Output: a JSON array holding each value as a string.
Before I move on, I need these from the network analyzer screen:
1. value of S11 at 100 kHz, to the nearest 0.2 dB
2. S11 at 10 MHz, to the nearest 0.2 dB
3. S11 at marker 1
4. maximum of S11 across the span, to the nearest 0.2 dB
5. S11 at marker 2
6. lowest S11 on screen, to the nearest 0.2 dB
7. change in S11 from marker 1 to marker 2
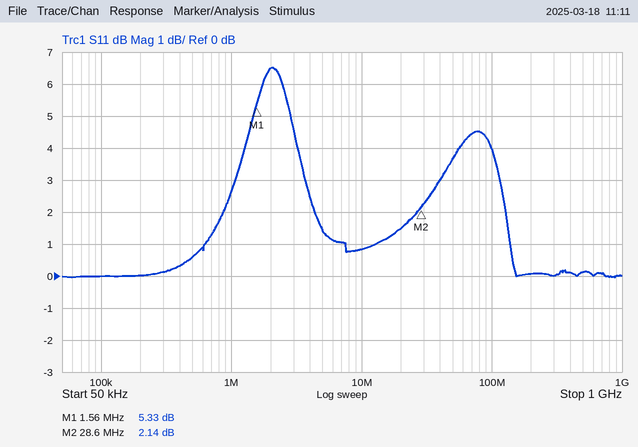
["0.0 dB", "0.8 dB", "5.33 dB", "6.6 dB", "2.14 dB", "0.0 dB", "-3.19 dB"]
